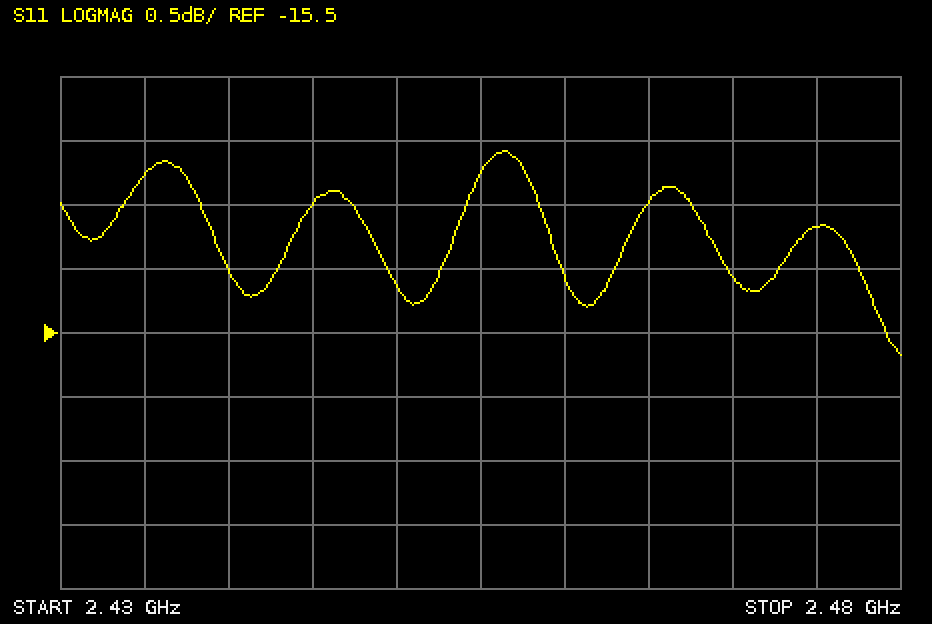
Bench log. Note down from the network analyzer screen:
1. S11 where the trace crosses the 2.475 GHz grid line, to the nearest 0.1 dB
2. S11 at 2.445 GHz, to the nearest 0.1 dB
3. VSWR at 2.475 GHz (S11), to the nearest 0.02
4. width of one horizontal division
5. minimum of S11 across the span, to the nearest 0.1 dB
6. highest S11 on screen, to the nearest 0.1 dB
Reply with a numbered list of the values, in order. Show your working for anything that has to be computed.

1. -14.7 dB
2. -14.5 dB
3. |Γ| = 10^(-14.7/20) = 0.1841; VSWR = (1 + 0.1841)/(1 − 0.1841) ≈ 1.45, so 1.46 to the nearest 0.02
4. 5 MHz
5. -15.7 dB
6. -14.1 dB
